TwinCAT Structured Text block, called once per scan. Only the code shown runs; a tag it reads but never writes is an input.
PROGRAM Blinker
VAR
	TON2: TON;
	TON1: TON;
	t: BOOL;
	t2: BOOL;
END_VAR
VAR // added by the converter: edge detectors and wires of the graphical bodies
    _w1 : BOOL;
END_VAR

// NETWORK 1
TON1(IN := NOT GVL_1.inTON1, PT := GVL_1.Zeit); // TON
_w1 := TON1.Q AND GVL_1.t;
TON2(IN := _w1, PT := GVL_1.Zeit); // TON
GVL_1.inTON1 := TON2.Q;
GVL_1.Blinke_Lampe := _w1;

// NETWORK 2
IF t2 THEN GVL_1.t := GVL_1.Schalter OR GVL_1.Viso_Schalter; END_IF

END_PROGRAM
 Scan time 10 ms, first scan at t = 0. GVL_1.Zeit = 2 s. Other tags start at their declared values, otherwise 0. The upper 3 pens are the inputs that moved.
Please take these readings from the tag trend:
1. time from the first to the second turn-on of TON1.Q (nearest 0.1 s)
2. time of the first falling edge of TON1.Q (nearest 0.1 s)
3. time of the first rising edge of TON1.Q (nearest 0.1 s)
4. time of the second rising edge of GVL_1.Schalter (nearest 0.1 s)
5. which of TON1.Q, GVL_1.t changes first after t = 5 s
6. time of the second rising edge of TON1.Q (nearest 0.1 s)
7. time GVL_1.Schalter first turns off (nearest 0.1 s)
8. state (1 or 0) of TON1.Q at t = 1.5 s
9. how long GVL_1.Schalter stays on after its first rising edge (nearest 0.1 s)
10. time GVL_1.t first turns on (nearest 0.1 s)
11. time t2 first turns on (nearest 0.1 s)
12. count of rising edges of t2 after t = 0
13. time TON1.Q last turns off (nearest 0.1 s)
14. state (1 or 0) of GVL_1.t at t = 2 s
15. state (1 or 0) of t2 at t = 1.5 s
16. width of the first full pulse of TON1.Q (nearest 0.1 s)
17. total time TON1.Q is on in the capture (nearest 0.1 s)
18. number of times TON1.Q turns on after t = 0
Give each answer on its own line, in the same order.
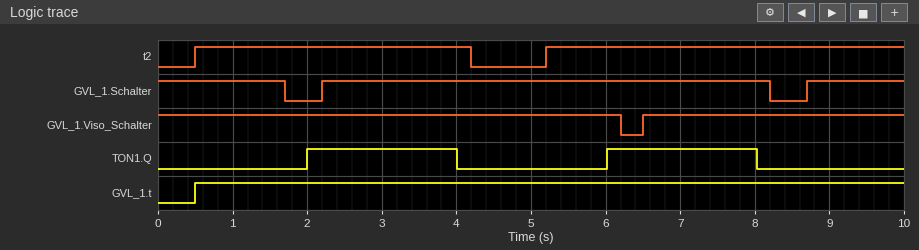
4.0 s
4.0 s
2.0 s
8.7 s
TON1.Q
6.0 s
1.7 s
0
6.0 s
0.5 s
0.5 s
2
8.0 s
1
1
2.0 s
4.0 s
2
